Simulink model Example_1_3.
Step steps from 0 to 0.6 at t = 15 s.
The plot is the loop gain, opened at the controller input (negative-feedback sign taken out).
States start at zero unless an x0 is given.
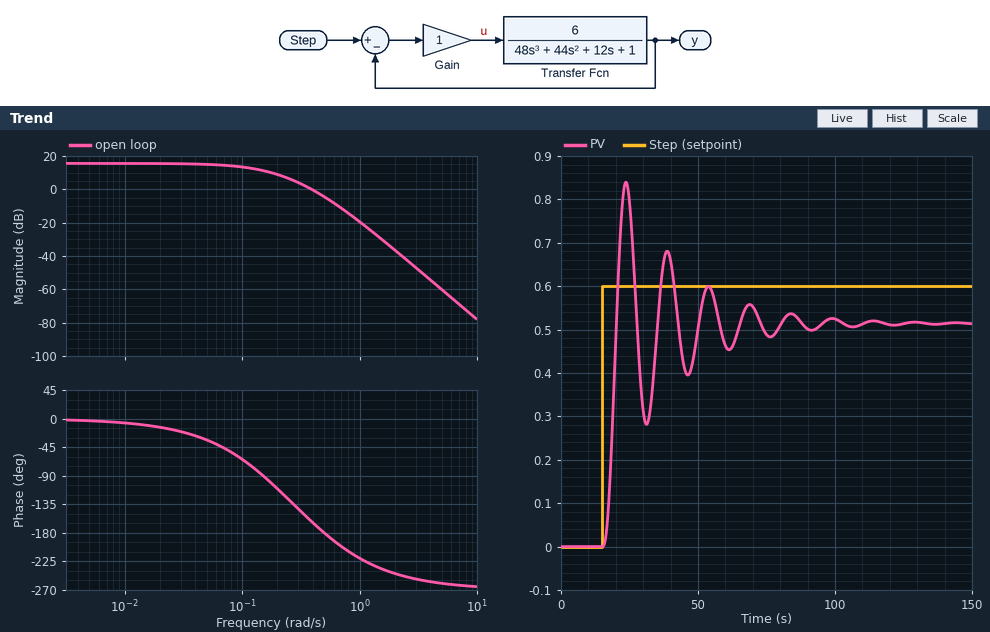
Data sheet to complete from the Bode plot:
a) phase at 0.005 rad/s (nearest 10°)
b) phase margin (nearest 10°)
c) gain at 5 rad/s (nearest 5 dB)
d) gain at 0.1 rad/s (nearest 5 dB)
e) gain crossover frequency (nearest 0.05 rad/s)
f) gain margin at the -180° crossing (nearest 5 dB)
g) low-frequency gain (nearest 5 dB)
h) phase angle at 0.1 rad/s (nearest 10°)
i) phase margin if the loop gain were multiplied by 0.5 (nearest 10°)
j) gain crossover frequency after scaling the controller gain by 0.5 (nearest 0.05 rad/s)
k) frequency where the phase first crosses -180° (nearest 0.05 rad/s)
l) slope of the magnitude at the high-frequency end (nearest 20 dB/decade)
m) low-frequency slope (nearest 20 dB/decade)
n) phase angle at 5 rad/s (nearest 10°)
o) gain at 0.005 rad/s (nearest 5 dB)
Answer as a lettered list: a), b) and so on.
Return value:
a) 0°
b) 20°
c) -60 dB
d) 15 dB
e) 0.40 rad/s
f) 5 dB
g) 15 dB
h) -60°
i) 50°
j) 0.25 rad/s
k) 0.50 rad/s
l) -60 dB/decade
m) 0 dB/decade
n) -260°
o) 15 dB
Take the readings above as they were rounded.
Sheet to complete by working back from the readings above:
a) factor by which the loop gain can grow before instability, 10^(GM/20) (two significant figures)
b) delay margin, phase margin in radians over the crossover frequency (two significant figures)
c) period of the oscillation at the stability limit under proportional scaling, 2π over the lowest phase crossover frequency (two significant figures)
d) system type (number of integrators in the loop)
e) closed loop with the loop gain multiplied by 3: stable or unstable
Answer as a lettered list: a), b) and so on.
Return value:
a) 1.8
b) 0.87 s
c) 13 s
d) 0
e) unstable
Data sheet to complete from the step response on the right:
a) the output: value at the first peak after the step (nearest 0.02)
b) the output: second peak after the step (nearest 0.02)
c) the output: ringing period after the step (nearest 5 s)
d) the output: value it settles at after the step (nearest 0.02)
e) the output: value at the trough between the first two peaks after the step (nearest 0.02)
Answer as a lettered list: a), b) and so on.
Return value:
a) 0.84
b) 0.68
c) 15 s
d) 0.52
e) 0.28
